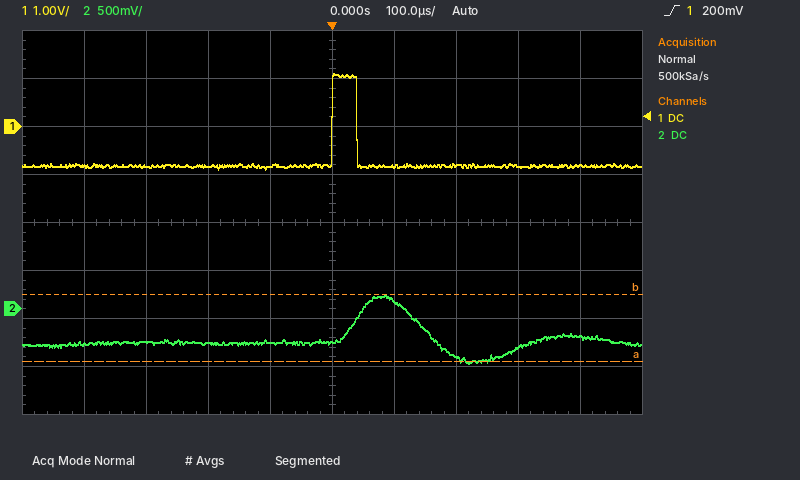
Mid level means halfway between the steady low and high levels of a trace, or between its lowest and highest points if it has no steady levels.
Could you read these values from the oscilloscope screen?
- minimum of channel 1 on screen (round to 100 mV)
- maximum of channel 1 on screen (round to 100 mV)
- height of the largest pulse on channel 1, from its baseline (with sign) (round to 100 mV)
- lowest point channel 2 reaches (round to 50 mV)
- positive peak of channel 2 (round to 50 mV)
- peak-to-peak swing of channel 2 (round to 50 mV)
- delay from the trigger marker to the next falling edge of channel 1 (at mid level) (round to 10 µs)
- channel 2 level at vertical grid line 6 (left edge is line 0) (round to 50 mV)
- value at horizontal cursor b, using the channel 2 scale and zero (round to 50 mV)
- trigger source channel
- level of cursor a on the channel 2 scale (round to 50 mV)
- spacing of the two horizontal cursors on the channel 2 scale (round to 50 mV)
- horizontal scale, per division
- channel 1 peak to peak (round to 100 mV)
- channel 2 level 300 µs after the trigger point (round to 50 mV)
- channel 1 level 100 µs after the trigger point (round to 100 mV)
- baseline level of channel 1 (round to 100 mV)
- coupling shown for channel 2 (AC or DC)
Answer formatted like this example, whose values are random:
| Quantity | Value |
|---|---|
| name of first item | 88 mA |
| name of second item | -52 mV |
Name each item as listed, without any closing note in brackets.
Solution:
| Quantity | Value |
|---|---|
| minimum of channel 1 on screen | -900 mV |
| maximum of channel 1 on screen | 1.1 V |
| height of the largest pulse on channel 1, from its baseline (with sign) | +1.9 V |
| lowest point channel 2 reaches | -550 mV |
| positive peak of channel 2 | 150 mV |
| peak-to-peak swing of channel 2 | 700 mV |
| delay from the trigger marker to the next falling edge of channel 1 (at mid level) | 40 µs |
| channel 2 level at vertical grid line 6 (left edge is line 0) | 100 mV |
| value at horizontal cursor b, using the channel 2 scale and zero | 150 mV |
| trigger source channel | channel 1 |
| level of cursor a on the channel 2 scale | -550 mV |
| spacing of the two horizontal cursors on the channel 2 scale | 700 mV |
| horizontal scale, per division | 100 µs |
| channel 1 peak to peak | 2.0 V |
| channel 2 level 300 µs after the trigger point | -400 mV |
| channel 1 level 100 µs after the trigger point | -800 mV |
| baseline level of channel 1 | -800 mV |
| coupling shown for channel 2 | DC |
